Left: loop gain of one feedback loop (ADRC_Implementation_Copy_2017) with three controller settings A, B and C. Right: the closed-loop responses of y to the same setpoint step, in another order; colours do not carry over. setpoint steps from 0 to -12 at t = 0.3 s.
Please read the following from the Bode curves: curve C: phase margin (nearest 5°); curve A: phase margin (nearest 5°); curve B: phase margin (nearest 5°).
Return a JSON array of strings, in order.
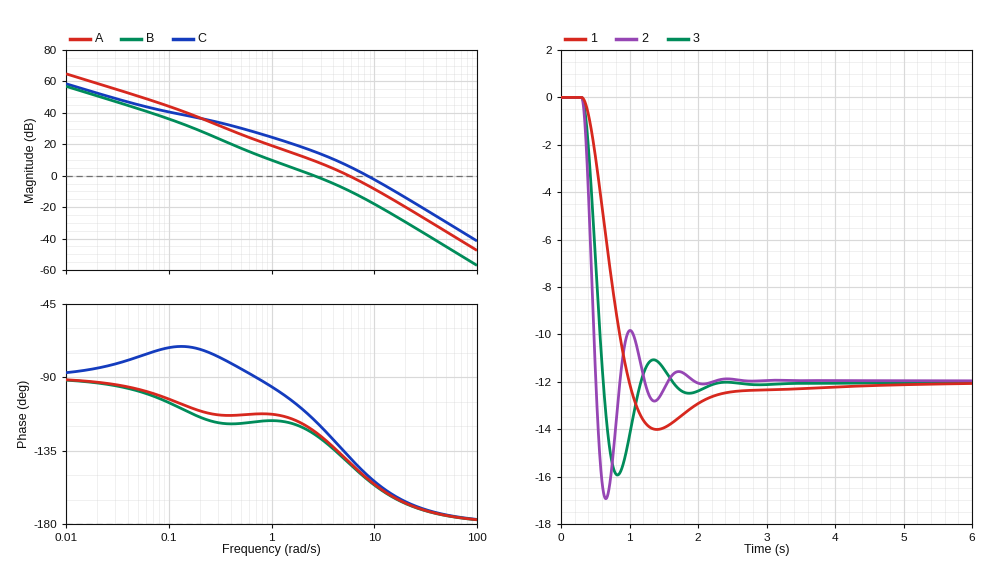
["30°", "40°", "55°"]
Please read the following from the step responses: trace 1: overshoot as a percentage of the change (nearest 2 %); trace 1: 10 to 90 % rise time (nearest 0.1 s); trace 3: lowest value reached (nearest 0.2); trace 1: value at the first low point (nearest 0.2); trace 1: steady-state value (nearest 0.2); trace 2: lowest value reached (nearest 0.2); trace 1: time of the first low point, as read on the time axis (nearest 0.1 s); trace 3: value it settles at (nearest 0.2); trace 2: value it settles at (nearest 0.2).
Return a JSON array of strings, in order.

["16 %", "0.5 s", "-16.0", "-14.0", "-12.0", "-17.0", "1.4 s", "-12.0", "-12.0"]
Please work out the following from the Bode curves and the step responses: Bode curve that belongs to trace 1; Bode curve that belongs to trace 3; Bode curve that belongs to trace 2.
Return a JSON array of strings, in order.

["B", "A", "C"]
